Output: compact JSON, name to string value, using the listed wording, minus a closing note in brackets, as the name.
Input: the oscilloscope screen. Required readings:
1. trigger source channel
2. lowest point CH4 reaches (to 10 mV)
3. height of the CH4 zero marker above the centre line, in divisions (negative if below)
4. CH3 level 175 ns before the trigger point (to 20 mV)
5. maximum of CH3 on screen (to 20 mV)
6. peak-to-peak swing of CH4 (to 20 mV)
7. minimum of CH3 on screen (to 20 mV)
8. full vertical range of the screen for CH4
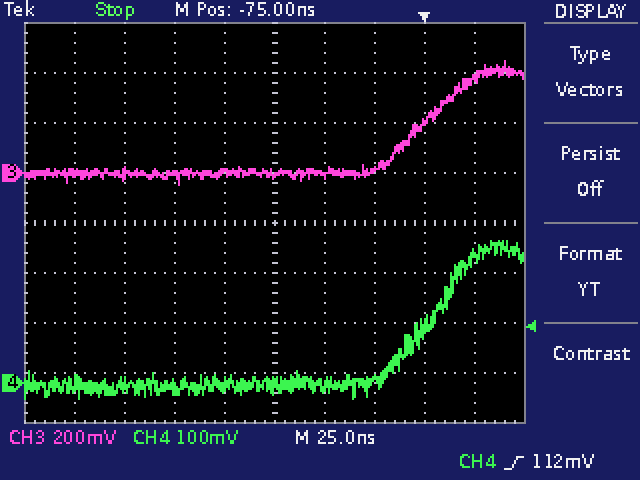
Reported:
{"trigger source channel": "CH4", "lowest point CH4 reaches": "-30 mV", "height of the CH4 zero marker above the centre line, in divisions": "-3.2 div", "CH3 level 175 ns before the trigger point": "0 mV", "maximum of CH3 on screen": "440 mV", "peak-to-peak swing of CH4": "320 mV", "minimum of CH3 on screen": "-40 mV", "full vertical range of the screen for CH4": "800 mV"}
